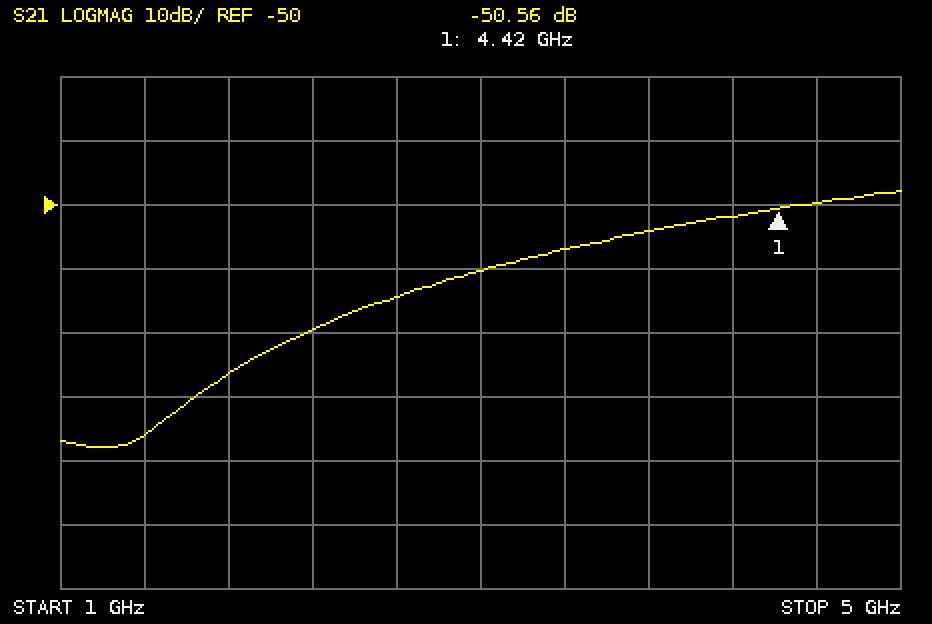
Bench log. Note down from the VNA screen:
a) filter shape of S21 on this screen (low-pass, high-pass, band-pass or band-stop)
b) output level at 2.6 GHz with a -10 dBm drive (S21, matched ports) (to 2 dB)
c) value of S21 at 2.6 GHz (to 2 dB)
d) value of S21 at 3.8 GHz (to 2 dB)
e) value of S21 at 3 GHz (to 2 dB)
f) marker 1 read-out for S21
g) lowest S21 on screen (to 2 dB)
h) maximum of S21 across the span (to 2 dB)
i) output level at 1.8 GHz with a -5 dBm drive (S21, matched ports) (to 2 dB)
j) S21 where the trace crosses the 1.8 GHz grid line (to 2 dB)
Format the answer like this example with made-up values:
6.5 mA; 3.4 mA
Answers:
high-pass; -74 dBm; -64 dB; -54 dB; -60 dB; -50.56 dB; -88 dB; -48 dB; -82 dBm; -76 dB
